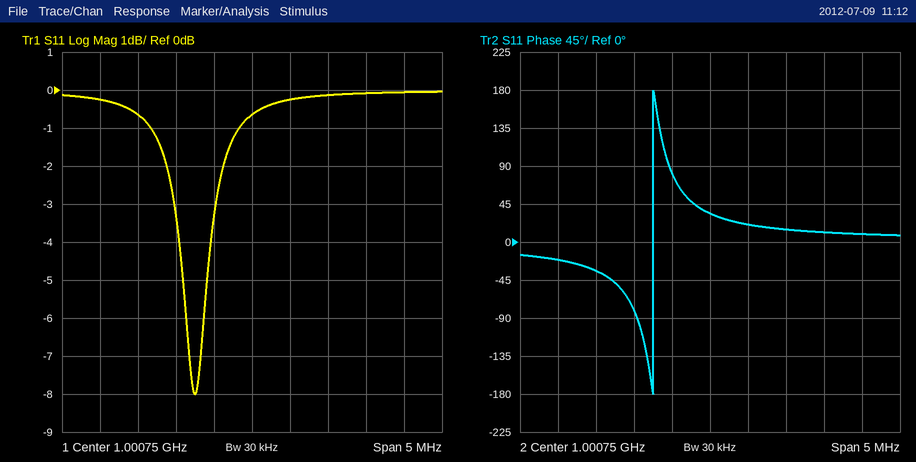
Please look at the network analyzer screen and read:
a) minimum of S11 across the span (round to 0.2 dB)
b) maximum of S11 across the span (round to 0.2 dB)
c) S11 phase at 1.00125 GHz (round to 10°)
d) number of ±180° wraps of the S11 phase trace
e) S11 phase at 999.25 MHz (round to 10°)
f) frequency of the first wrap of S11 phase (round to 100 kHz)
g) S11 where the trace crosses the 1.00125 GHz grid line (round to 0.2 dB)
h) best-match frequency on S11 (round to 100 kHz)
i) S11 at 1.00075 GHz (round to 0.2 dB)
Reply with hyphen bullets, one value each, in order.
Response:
- -8.0 dB
- 0.0 dB
- 20°
- 1
- -30°
- 1.0000 GHz
- -0.2 dB
- 1.0000 GHz
- -0.6 dB
